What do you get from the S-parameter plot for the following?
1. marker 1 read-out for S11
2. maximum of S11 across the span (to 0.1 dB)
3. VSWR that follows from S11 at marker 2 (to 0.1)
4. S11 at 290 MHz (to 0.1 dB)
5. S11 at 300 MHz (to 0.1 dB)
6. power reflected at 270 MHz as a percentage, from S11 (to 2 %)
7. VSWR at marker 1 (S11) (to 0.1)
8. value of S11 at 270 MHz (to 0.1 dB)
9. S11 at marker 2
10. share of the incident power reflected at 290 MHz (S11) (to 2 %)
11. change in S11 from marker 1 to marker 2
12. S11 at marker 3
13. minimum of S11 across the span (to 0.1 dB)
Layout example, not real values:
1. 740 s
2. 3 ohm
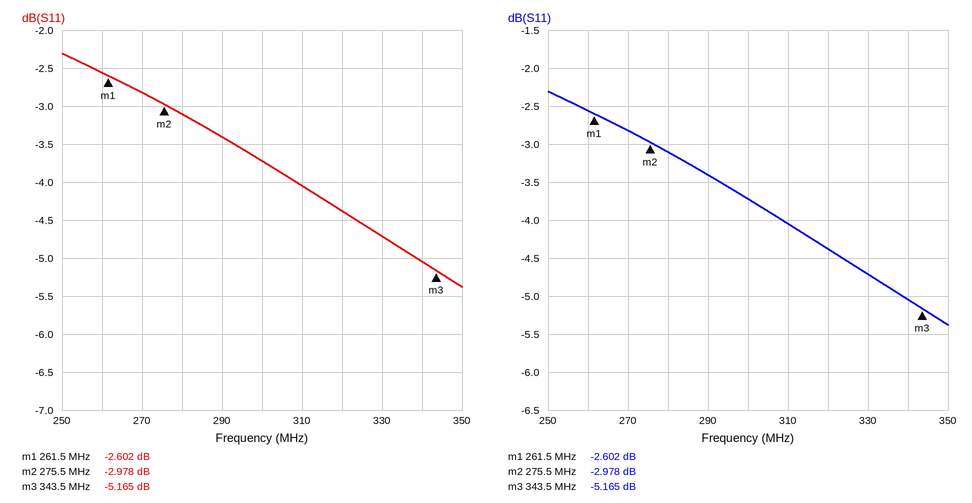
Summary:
1. -2.602 dB
2. -2.3 dB
3. 5.9
4. -3.4 dB
5. -3.7 dB
6. 52 %
7. 6.7
8. -2.8 dB
9. -2.978 dB
10. 46 %
11. -0.376 dB
12. -5.165 dB
13. -5.4 dB
